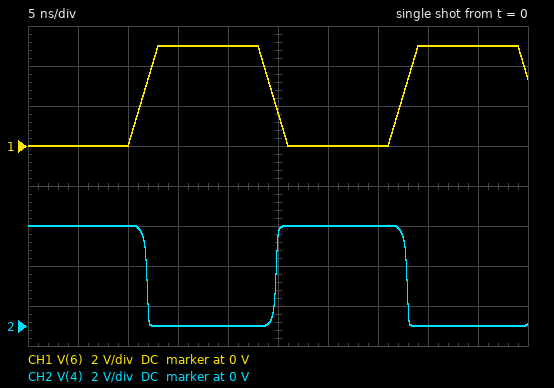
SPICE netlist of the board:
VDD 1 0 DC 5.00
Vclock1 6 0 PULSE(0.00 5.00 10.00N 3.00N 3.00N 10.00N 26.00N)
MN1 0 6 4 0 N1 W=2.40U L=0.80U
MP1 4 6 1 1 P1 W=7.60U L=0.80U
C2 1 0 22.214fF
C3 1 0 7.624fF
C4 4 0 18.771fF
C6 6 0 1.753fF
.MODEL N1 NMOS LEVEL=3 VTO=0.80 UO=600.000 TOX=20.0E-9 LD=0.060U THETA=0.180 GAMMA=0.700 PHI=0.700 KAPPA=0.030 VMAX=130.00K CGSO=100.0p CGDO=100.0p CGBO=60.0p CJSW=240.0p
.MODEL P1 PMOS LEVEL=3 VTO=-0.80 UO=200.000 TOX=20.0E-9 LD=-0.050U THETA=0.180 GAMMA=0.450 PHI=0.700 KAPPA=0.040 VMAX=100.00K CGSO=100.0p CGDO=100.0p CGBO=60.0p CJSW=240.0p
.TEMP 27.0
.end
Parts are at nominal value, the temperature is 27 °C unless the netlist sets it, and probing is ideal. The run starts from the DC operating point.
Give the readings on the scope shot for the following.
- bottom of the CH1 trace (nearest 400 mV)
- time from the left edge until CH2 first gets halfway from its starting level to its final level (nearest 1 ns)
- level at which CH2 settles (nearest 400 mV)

0 V
12 ns
0 V
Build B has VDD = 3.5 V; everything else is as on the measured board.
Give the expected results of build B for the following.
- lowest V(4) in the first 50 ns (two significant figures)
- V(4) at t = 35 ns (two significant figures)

-7.6 mV
3.5 V
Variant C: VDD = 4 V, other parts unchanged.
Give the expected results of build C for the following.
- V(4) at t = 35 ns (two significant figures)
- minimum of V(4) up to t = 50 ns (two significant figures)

4.0 V
-6.5 mV
